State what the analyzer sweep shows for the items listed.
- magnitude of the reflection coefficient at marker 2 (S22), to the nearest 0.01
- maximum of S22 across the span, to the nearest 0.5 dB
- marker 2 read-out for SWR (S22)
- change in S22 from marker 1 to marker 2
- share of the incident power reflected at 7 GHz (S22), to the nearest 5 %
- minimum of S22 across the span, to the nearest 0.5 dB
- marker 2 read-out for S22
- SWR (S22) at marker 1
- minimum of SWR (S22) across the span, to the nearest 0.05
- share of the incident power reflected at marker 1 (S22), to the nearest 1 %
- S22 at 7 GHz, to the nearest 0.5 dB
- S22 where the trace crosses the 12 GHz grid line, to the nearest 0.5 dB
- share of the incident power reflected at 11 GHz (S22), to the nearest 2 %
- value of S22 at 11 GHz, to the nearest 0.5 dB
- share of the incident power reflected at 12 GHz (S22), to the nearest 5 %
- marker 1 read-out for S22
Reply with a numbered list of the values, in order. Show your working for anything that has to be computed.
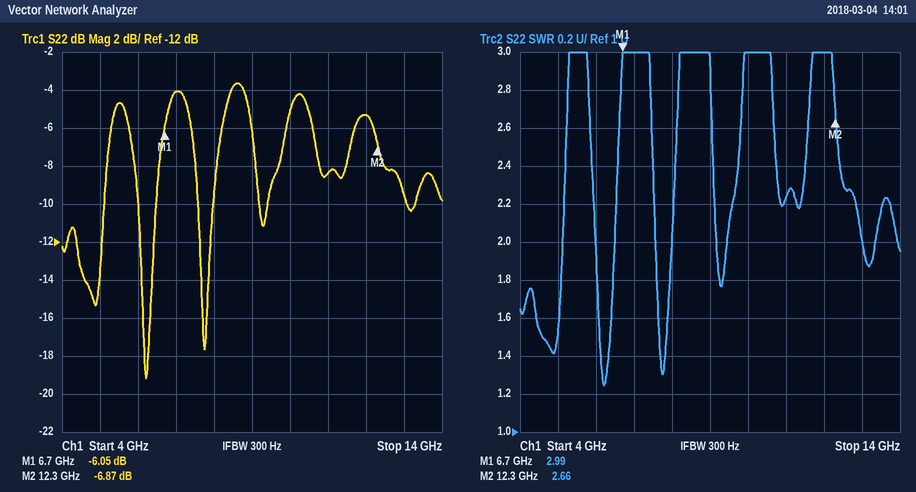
1. 10^(-6.87/20) ≈ 0.45
2. -3.5 dB
3. 2.66
4. -6.87 − (-6.05) = -0.82 dB
5. 10^(-4/10) ≈ 40 %
6. -19.0 dB
7. -6.87 dB
8. 2.99
9. 1.25
10. 10^(-6.05/10) ≈ 25 %
11. -4.0 dB
12. -5.5 dB
13. 10^(-8.5/10) ≈ 14 %
14. -8.5 dB
15. 10^(-5.5/10) ≈ 28.2 %, so 30 % to the nearest 5 %
16. -6.05 dB
